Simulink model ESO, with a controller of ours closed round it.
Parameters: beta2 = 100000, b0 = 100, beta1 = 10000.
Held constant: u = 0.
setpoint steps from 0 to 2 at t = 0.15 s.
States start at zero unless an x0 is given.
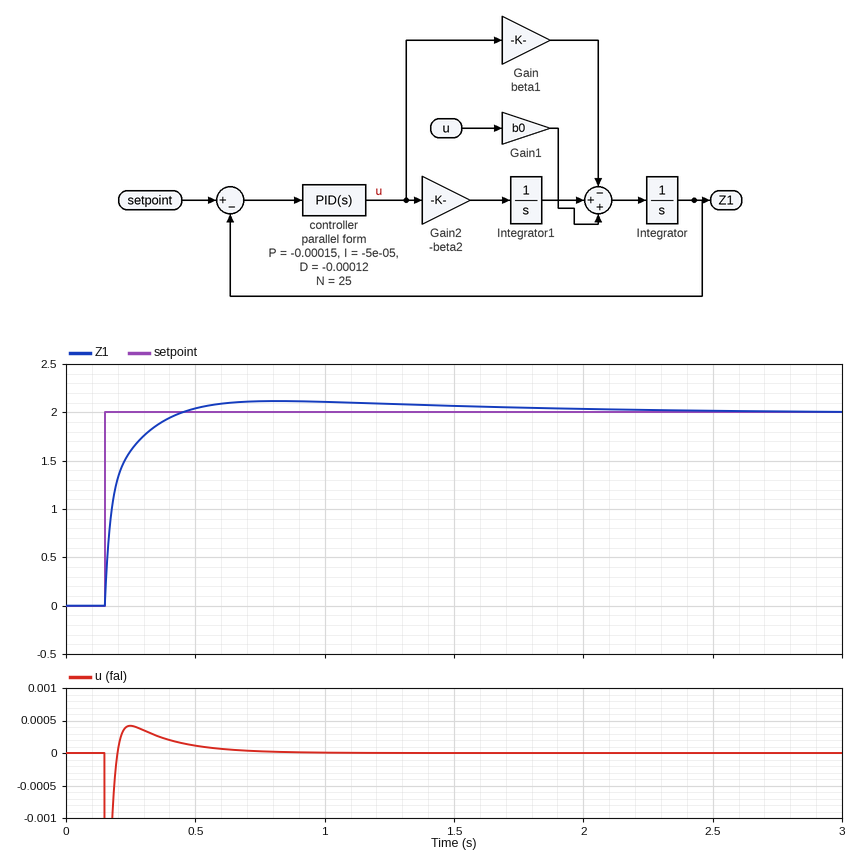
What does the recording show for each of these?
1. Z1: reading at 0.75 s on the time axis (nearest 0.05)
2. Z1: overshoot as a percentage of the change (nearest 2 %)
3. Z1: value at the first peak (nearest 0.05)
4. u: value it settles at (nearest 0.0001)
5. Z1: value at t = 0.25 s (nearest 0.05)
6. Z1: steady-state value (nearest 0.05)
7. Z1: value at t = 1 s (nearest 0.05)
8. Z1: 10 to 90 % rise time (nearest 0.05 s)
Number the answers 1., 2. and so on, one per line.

1. 2.10
2. 6 %
3. 2.10
4. 0.0000
5. 1.60
6. 2.00
7. 2.10
8. 0.15 s
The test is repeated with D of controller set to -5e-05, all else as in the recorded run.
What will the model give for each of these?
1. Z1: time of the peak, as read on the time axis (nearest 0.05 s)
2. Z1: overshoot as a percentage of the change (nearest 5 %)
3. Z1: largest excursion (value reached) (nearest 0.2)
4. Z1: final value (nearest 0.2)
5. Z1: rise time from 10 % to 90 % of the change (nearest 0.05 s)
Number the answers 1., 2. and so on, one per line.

1. 0.80 s
2. 15 %
3. 2.4
4. 2.0
5. 0.25 s
